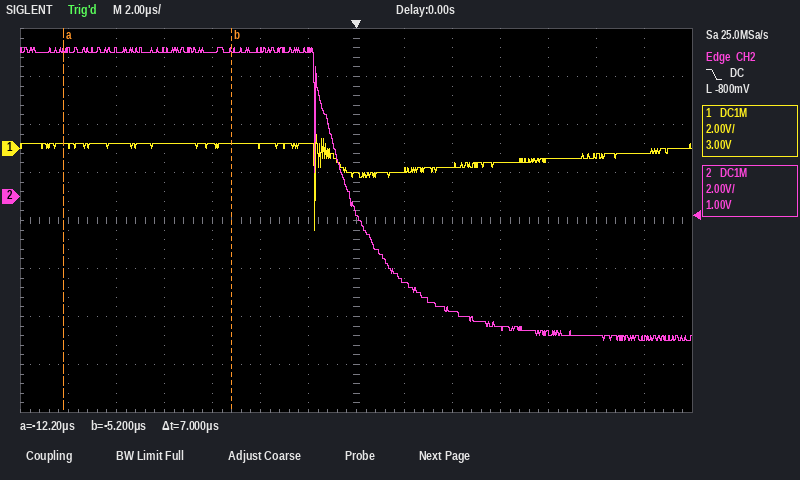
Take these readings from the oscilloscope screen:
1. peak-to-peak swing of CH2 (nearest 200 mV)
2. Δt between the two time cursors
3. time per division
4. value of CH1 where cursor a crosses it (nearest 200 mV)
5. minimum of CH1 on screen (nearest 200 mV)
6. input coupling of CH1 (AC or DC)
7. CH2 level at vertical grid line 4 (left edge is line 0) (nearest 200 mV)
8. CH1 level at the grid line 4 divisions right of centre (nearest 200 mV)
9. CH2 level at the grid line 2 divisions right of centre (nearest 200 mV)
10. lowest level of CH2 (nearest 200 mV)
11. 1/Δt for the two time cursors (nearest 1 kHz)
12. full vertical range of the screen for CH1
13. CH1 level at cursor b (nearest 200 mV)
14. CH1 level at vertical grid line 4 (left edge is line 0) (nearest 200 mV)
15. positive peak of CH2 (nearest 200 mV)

12.2 V
7 µs
2 µs
200 mV
-3.4 V
DC
6.0 V
-400 mV
-4.8 V
-6.0 V
143 kHz
16 V
200 mV
200 mV
6.2 V
